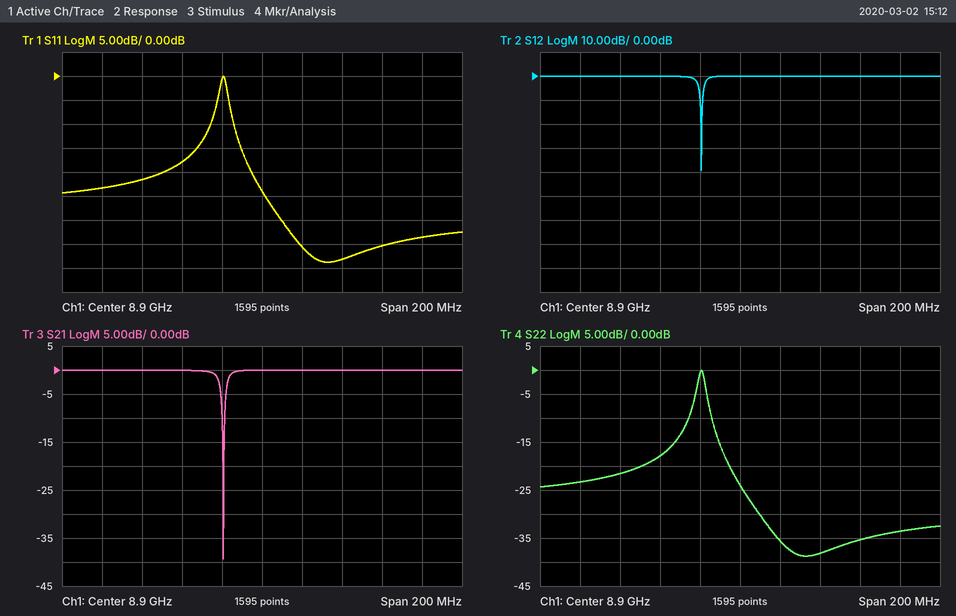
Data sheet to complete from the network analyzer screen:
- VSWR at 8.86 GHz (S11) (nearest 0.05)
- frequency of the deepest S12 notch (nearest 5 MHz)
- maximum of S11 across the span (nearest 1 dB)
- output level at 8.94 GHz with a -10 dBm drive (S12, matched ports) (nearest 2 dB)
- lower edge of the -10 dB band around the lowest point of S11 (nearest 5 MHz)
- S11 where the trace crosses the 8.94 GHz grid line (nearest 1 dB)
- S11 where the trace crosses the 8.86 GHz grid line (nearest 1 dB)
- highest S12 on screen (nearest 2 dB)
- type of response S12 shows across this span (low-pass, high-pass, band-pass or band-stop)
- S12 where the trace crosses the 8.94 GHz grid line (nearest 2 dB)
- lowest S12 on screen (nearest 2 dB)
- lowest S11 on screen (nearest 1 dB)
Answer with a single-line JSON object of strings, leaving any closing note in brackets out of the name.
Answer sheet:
{"VSWR at 8.86 GHz (S11)": "1.30", "frequency of the deepest S12 notch": "8.880 GHz", "maximum of S11 across the span": "0 dB", "output level at 8.94 GHz with a -10 dBm drive (S12, matched ports)": "-10 dBm", "lower edge of the -10 dB band around the lowest point of S11": "8.885 GHz", "S11 where the trace crosses the 8.94 GHz grid line": "-38 dB", "S11 where the trace crosses the 8.86 GHz grid line": "-18 dB", "highest S12 on screen": "0 dB", "type of response S12 shows across this span": "band-stop", "S12 where the trace crosses the 8.94 GHz grid line": "0 dB", "lowest S12 on screen": "-40 dB", "lowest S11 on screen": "-39 dB"}
